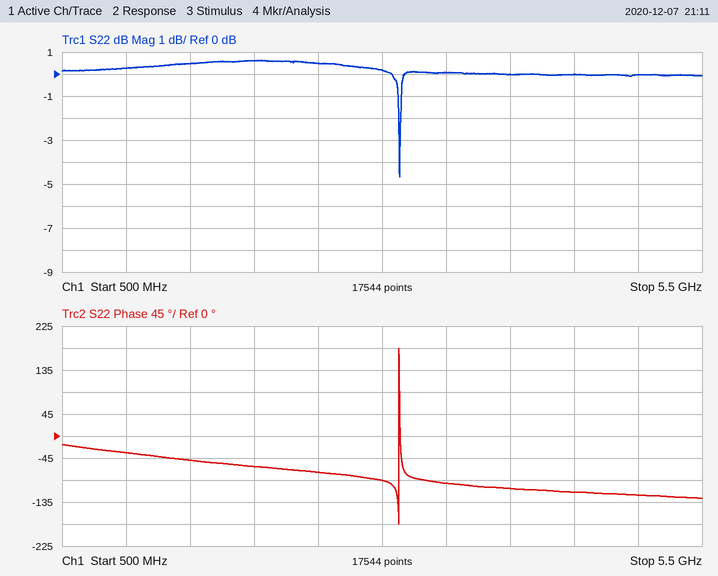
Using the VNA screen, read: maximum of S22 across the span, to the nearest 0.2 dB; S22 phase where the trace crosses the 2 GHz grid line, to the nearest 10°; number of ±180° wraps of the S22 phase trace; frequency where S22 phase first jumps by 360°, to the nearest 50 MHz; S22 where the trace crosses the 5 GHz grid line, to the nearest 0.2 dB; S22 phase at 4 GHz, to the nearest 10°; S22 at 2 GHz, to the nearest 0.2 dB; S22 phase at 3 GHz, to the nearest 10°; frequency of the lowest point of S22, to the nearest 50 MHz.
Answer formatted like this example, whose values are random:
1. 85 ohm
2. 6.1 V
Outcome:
1. 0.6 dB
2. -60°
3. 1
4. 3.15 GHz
5. 0.0 dB
6. -110°
7. 0.6 dB
8. -90°
9. 3.15 GHz
